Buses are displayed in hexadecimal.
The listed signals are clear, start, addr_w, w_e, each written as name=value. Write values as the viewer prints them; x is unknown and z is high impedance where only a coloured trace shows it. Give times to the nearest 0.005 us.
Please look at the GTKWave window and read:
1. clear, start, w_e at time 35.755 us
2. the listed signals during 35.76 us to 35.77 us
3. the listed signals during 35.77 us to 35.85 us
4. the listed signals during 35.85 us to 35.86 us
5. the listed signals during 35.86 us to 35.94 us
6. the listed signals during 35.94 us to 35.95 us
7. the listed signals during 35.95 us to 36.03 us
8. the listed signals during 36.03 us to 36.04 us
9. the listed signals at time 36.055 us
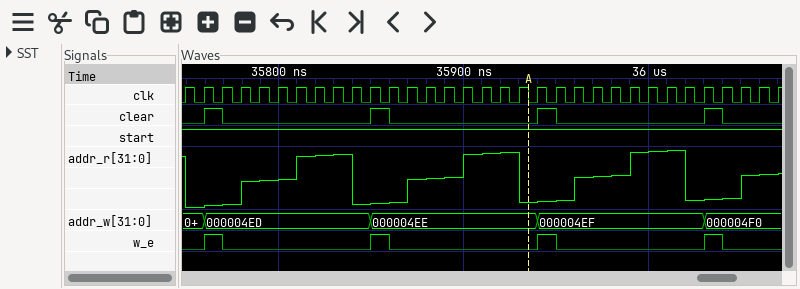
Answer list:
clear=0, start=1, w_e=0
clear=1, start=1, addr_w=000004ED, w_e=1
clear=0, start=1, addr_w=000004ED, w_e=0
clear=1, start=1, addr_w=000004EE, w_e=1
clear=0, start=1, addr_w=000004EE, w_e=0
clear=1, start=1, addr_w=000004EF, w_e=1
clear=0, start=1, addr_w=000004EF, w_e=0
clear=1, start=1, addr_w=000004F0, w_e=1
clear=0, start=1, addr_w=000004F0, w_e=0
